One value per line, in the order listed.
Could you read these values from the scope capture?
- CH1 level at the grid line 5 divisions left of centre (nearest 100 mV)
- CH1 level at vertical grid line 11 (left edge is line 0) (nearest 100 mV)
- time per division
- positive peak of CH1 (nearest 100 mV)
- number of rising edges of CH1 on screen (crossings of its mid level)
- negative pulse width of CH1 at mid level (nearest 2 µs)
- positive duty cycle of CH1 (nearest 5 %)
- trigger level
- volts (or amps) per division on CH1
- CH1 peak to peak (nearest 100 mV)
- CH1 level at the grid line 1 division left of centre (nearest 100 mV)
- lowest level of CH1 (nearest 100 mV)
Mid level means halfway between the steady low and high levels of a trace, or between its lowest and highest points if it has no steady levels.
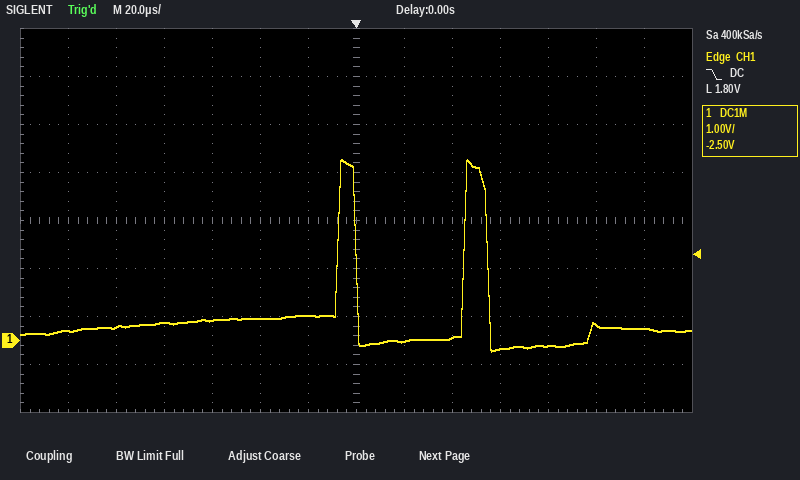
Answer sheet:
300 mV
-100 mV
20 µs
3.8 V
2
44 µs
15 %
1.80 V
1 V
4.0 V
500 mV
-200 mV
